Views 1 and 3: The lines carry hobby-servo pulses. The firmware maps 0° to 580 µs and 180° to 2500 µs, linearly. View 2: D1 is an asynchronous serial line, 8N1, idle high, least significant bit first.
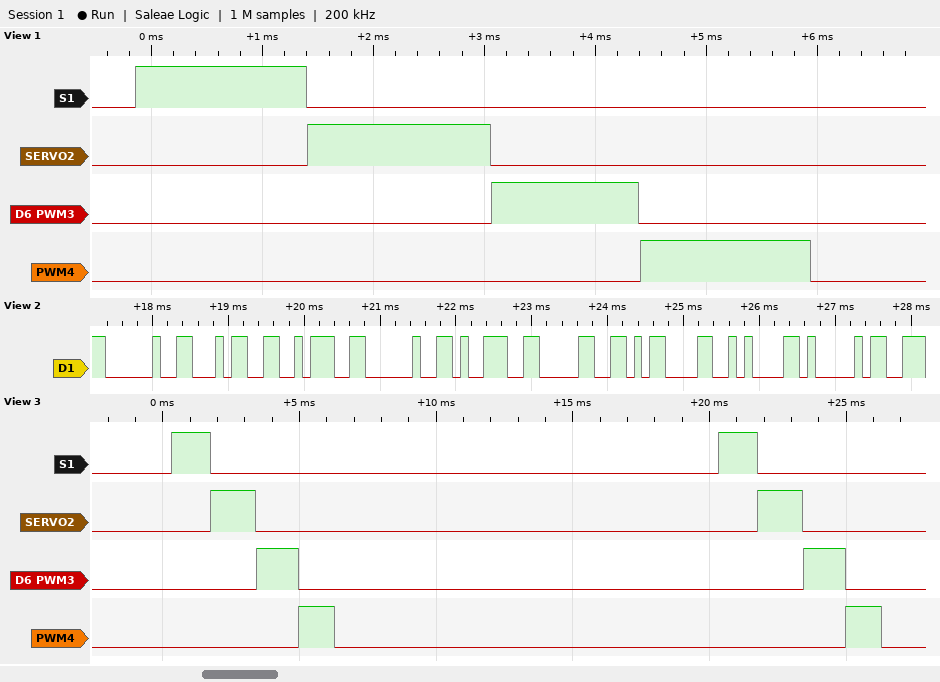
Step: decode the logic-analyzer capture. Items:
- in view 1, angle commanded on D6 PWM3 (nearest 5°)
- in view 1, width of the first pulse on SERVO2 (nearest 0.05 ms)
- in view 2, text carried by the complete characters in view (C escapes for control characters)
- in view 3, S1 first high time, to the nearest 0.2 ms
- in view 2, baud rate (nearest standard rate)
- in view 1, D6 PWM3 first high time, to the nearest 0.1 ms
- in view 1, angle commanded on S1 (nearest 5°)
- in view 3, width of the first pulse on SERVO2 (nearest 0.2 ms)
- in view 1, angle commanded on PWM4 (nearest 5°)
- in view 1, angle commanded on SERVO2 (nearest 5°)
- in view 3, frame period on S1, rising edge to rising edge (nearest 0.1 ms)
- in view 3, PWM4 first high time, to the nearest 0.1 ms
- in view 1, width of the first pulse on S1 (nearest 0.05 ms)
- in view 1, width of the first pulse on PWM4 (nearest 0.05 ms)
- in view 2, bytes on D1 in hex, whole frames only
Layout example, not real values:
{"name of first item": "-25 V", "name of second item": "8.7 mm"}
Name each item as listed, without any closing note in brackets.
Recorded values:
{"in view 1, angle commanded on D6 PWM3": "70°", "in view 1, width of the first pulse on SERVO2": "1.65 ms", "in view 2, text carried by the complete characters in view": "\" 4: 90\\r\\nA\"", "in view 3, S1 first high time, to the nearest 0.2 ms": "1.4 ms", "in view 2, baud rate": "9600 baud", "in view 1, D6 PWM3 first high time, to the nearest 0.1 ms": "1.3 ms", "in view 1, angle commanded on S1": "90°", "in view 3, width of the first pulse on SERVO2": "1.6 ms", "in view 1, angle commanded on PWM4": "90°", "in view 1, angle commanded on SERVO2": "100°", "in view 3, frame period on S1, rising edge to rising edge": "20.0 ms", "in view 3, PWM4 first high time, to the nearest 0.1 ms": "1.3 ms", "in view 1, width of the first pulse on S1": "1.55 ms", "in view 1, width of the first pulse on PWM4": "1.55 ms", "in view 2, bytes on D1 in hex, whole frames only": "20 34 3A 20 39 30 0D 0A 41"}
